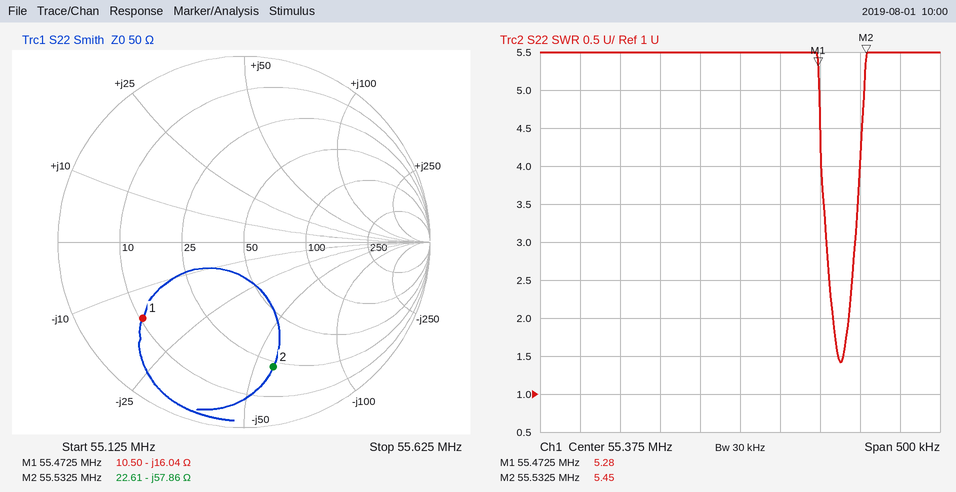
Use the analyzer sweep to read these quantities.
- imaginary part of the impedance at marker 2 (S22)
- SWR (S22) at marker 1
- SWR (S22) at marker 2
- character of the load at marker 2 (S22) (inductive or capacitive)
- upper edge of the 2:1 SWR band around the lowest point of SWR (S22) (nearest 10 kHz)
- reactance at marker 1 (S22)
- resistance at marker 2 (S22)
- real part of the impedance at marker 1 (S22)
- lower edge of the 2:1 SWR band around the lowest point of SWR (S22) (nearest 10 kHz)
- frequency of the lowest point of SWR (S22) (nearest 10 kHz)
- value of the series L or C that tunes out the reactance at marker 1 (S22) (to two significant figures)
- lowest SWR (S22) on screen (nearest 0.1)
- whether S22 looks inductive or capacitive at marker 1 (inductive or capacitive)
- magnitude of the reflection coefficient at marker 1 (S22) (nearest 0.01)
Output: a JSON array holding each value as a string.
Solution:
["-57.86 Ω", "5.28", "5.45", "capacitive", "55.51 MHz", "-16.04 Ω", "22.61 Ω", "10.50 Ω", "55.49 MHz", "55.50 MHz", "46 nH", "1.4", "capacitive", "0.68"]
